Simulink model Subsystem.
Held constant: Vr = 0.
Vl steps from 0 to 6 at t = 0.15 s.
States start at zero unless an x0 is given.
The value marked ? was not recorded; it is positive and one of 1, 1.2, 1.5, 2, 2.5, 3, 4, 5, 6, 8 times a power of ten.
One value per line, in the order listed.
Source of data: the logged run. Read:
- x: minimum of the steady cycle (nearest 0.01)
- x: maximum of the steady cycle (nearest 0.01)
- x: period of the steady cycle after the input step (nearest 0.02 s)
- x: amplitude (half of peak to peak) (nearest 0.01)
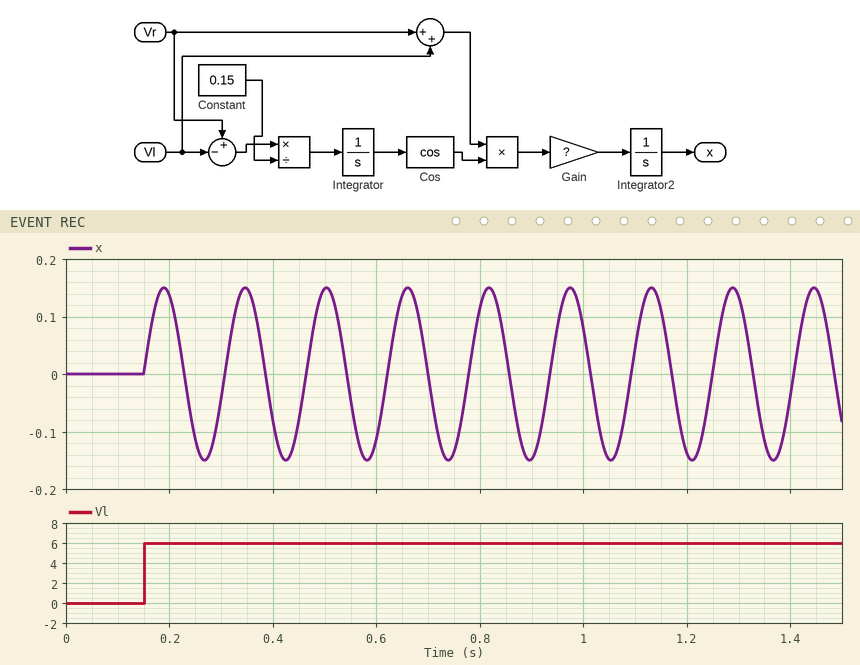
-0.15
0.15
0.16 s
0.15
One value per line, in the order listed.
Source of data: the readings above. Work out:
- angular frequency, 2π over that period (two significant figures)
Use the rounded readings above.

39 rad/s
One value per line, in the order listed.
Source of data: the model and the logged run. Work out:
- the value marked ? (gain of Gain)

1
